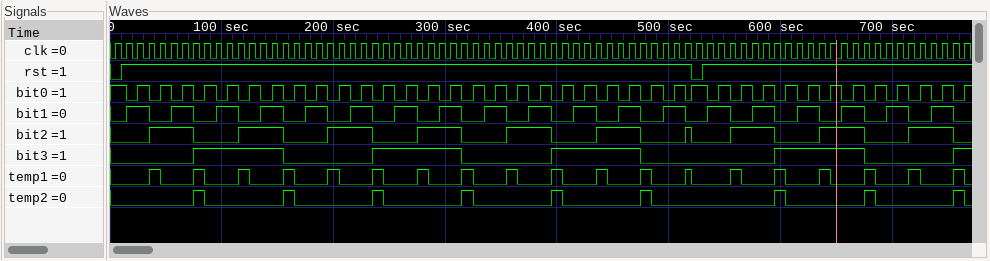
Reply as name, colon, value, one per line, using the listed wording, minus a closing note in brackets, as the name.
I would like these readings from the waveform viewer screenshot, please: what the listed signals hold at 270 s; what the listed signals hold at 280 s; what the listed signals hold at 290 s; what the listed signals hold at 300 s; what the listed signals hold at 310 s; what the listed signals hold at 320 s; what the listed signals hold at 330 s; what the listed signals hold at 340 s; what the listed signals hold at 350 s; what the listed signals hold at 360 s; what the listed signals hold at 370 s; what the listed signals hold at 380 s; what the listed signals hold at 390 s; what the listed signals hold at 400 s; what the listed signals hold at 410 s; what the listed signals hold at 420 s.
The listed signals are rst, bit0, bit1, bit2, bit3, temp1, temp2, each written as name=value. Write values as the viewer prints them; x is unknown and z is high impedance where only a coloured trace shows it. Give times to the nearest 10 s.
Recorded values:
what the listed signals hold at 270 s: rst=1, bit0=1, bit1=1, bit2=0, bit3=1, temp1=0, temp2=0
what the listed signals hold at 280 s: rst=1, bit0=0, bit1=0, bit2=1, bit3=1, temp1=1, temp2=0
what the listed signals hold at 290 s: rst=1, bit0=1, bit1=0, bit2=1, bit3=1, temp1=0, temp2=0
what the listed signals hold at 300 s: rst=1, bit0=0, bit1=1, bit2=1, bit3=1, temp1=0, temp2=0
what the listed signals hold at 310 s: rst=1, bit0=1, bit1=1, bit2=1, bit3=1, temp1=0, temp2=0
what the listed signals hold at 320 s: rst=1, bit0=0, bit1=0, bit2=0, bit3=0, temp1=1, temp2=1
what the listed signals hold at 330 s: rst=1, bit0=1, bit1=0, bit2=0, bit3=0, temp1=0, temp2=0
what the listed signals hold at 340 s: rst=1, bit0=0, bit1=1, bit2=0, bit3=0, temp1=0, temp2=0
what the listed signals hold at 350 s: rst=1, bit0=1, bit1=1, bit2=0, bit3=0, temp1=0, temp2=0
what the listed signals hold at 360 s: rst=1, bit0=0, bit1=0, bit2=1, bit3=0, temp1=1, temp2=0
what the listed signals hold at 370 s: rst=1, bit0=1, bit1=0, bit2=1, bit3=0, temp1=0, temp2=0
what the listed signals hold at 380 s: rst=1, bit0=0, bit1=1, bit2=1, bit3=0, temp1=0, temp2=0
what the listed signals hold at 390 s: rst=1, bit0=1, bit1=1, bit2=1, bit3=0, temp1=0, temp2=0
what the listed signals hold at 400 s: rst=1, bit0=0, bit1=0, bit2=0, bit3=1, temp1=1, temp2=1
what the listed signals hold at 410 s: rst=1, bit0=1, bit1=0, bit2=0, bit3=1, temp1=0, temp2=0
what the listed signals hold at 420 s: rst=1, bit0=0, bit1=1, bit2=0, bit3=1, temp1=0, temp2=0
